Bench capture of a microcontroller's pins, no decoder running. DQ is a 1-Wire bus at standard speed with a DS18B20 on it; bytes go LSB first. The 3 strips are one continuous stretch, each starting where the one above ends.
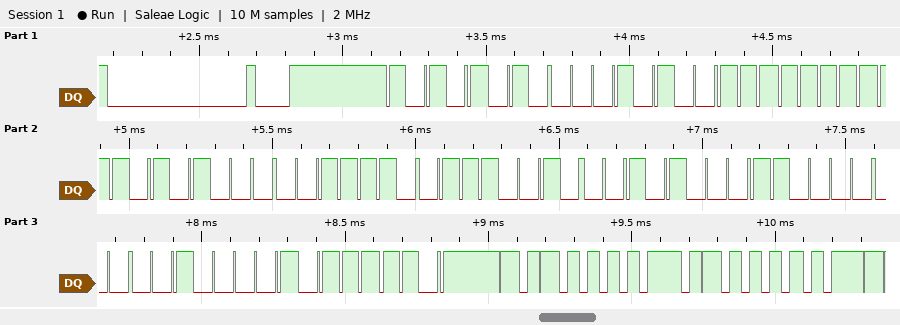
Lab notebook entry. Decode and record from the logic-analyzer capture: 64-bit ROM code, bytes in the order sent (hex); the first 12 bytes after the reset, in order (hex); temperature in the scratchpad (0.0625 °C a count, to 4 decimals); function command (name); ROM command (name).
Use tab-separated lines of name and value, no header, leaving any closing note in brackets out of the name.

64-bit ROM code, bytes in the order sent	28 FF 2B 78 4E 14 03 84
the first 12 bytes after the reset, in order	55 28 FF 2B 78 4E 14 03 84 BE 05 02
temperature in the scratchpad	32.3125 °C
function command	Read Scratchpad
ROM command	Match ROM
